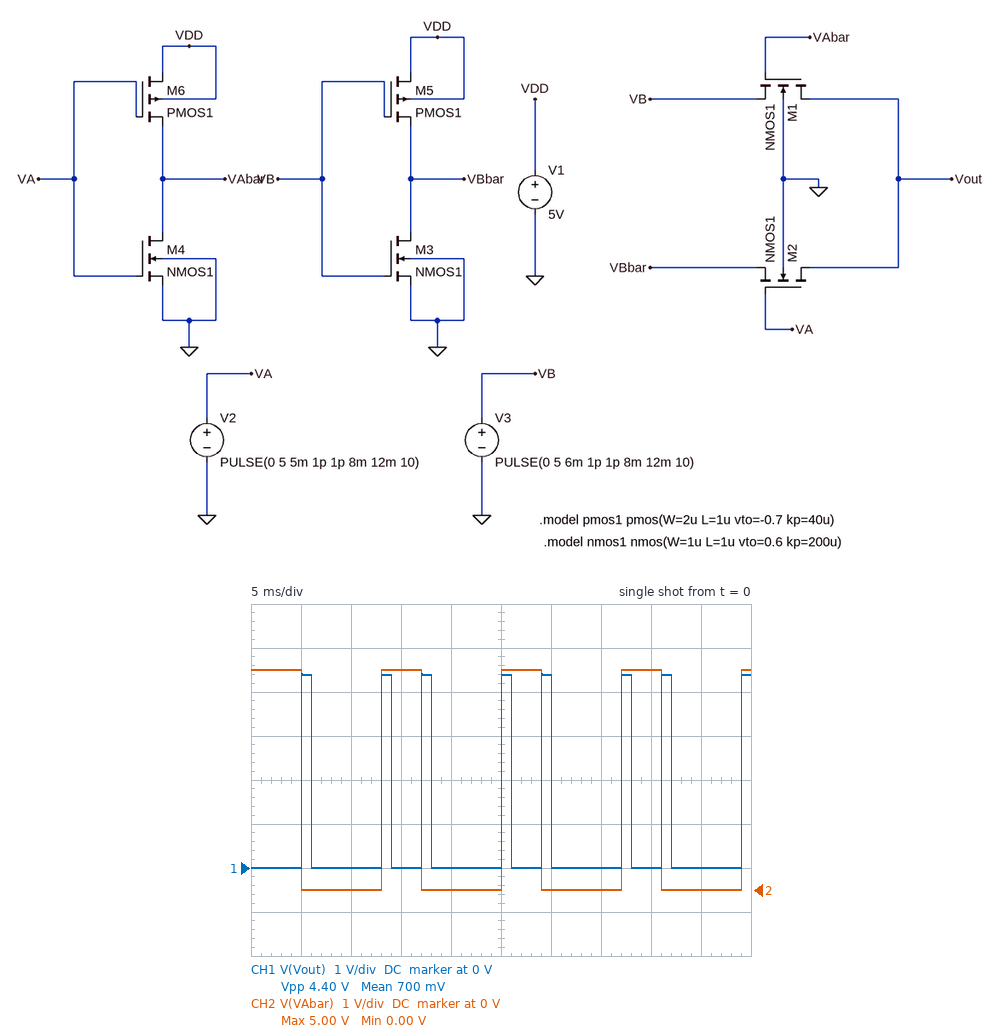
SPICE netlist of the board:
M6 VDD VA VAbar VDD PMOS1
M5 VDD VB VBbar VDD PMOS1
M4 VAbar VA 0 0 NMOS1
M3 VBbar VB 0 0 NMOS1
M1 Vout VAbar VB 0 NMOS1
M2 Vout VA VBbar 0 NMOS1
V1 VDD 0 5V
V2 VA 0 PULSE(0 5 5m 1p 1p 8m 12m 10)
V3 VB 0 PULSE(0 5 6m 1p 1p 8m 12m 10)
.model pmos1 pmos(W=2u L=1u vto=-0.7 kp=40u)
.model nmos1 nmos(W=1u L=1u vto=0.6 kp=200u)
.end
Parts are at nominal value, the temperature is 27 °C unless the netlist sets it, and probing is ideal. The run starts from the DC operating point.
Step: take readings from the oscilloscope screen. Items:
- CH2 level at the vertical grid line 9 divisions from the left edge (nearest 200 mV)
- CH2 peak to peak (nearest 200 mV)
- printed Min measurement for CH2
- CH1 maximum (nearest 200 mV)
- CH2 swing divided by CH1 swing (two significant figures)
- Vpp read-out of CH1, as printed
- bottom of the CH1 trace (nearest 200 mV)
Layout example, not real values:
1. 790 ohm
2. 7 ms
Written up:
1. 0 V
2. 5.0 V
3. 0.00 V
4. 4.4 V
5. 1.1
6. 4.40 V
7. 0 V
